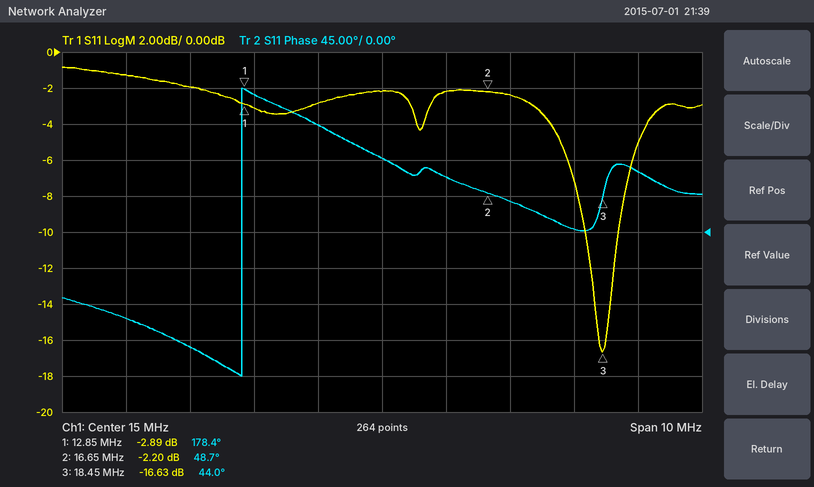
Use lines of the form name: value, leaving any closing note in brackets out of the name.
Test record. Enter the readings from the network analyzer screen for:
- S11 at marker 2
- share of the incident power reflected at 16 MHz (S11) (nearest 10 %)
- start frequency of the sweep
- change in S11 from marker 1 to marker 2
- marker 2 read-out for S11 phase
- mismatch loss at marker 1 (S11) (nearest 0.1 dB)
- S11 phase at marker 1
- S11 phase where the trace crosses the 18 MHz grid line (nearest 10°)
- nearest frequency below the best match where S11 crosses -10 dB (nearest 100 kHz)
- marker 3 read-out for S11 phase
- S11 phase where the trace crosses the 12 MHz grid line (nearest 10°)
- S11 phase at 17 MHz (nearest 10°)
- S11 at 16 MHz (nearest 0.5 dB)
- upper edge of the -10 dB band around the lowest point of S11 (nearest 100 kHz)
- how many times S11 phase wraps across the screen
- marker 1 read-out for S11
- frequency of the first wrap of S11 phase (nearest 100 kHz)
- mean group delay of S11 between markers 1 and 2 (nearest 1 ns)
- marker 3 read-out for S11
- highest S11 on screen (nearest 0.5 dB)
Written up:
S11 at marker 2: -2.20 dB
share of the incident power reflected at 16 MHz (S11): 60 %
start frequency of the sweep: 10 MHz
change in S11 from marker 1 to marker 2: 0.69 dB
marker 2 read-out for S11 phase: 48.7°
mismatch loss at marker 1 (S11): 3.1 dB
S11 phase at marker 1: 178.4°
S11 phase where the trace crosses the 18 MHz grid line: 0°
nearest frequency below the best match where S11 crosses -10 dB: 18.2 MHz
marker 3 read-out for S11 phase: 44.0°
S11 phase where the trace crosses the 12 MHz grid line: -140°
S11 phase at 17 MHz: 40°
S11 at 16 MHz: -2.0 dB
upper edge of the -10 dB band around the lowest point of S11: 18.7 MHz
how many times S11 phase wraps across the screen: 1
marker 1 read-out for S11: -2.89 dB
frequency of the first wrap of S11 phase: 12.8 MHz
mean group delay of S11 between markers 1 and 2: 95 ns
marker 3 read-out for S11: -16.63 dB
highest S11 on screen: -1.0 dB
